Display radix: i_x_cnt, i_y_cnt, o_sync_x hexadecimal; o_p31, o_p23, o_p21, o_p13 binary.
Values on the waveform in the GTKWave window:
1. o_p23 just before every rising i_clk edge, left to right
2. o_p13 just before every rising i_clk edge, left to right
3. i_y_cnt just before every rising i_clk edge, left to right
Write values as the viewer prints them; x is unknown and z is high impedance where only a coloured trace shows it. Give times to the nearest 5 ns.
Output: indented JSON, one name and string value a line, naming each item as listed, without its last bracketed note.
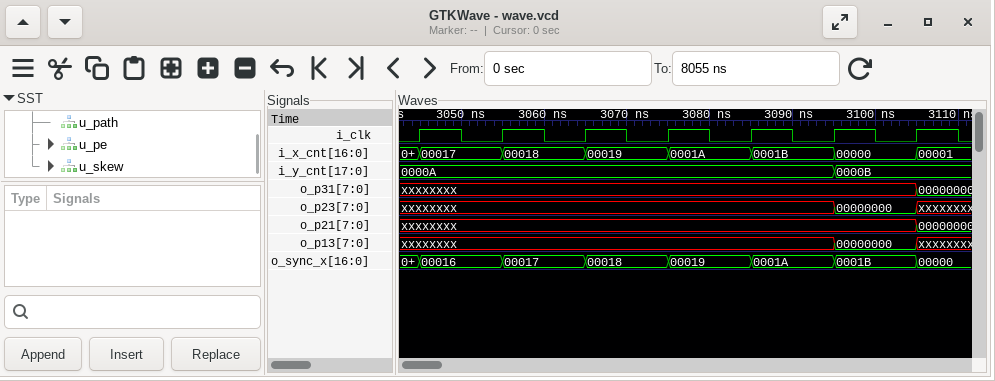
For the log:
{
  "o_p23 just before every rising i_clk edge, left to right": "xxxxxxxx, xxxxxxxx, xxxxxxxx, xxxxxxxx, xxxxxxxx, xxxxxxxx, 00000000",
  "o_p13 just before every rising i_clk edge, left to right": "xxxxxxxx, xxxxxxxx, xxxxxxxx, xxxxxxxx, xxxxxxxx, xxxxxxxx, 00000000",
  "i_y_cnt just before every rising i_clk edge, left to right": "0000A, 0000A, 0000A, 0000A, 0000A, 0000A, 0000B"
}
